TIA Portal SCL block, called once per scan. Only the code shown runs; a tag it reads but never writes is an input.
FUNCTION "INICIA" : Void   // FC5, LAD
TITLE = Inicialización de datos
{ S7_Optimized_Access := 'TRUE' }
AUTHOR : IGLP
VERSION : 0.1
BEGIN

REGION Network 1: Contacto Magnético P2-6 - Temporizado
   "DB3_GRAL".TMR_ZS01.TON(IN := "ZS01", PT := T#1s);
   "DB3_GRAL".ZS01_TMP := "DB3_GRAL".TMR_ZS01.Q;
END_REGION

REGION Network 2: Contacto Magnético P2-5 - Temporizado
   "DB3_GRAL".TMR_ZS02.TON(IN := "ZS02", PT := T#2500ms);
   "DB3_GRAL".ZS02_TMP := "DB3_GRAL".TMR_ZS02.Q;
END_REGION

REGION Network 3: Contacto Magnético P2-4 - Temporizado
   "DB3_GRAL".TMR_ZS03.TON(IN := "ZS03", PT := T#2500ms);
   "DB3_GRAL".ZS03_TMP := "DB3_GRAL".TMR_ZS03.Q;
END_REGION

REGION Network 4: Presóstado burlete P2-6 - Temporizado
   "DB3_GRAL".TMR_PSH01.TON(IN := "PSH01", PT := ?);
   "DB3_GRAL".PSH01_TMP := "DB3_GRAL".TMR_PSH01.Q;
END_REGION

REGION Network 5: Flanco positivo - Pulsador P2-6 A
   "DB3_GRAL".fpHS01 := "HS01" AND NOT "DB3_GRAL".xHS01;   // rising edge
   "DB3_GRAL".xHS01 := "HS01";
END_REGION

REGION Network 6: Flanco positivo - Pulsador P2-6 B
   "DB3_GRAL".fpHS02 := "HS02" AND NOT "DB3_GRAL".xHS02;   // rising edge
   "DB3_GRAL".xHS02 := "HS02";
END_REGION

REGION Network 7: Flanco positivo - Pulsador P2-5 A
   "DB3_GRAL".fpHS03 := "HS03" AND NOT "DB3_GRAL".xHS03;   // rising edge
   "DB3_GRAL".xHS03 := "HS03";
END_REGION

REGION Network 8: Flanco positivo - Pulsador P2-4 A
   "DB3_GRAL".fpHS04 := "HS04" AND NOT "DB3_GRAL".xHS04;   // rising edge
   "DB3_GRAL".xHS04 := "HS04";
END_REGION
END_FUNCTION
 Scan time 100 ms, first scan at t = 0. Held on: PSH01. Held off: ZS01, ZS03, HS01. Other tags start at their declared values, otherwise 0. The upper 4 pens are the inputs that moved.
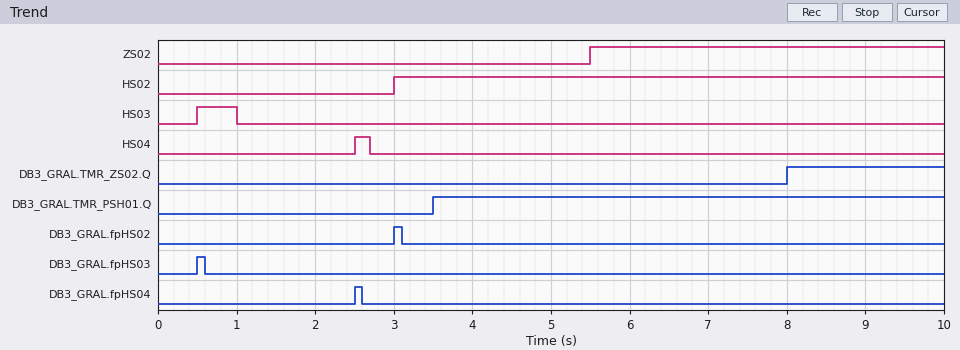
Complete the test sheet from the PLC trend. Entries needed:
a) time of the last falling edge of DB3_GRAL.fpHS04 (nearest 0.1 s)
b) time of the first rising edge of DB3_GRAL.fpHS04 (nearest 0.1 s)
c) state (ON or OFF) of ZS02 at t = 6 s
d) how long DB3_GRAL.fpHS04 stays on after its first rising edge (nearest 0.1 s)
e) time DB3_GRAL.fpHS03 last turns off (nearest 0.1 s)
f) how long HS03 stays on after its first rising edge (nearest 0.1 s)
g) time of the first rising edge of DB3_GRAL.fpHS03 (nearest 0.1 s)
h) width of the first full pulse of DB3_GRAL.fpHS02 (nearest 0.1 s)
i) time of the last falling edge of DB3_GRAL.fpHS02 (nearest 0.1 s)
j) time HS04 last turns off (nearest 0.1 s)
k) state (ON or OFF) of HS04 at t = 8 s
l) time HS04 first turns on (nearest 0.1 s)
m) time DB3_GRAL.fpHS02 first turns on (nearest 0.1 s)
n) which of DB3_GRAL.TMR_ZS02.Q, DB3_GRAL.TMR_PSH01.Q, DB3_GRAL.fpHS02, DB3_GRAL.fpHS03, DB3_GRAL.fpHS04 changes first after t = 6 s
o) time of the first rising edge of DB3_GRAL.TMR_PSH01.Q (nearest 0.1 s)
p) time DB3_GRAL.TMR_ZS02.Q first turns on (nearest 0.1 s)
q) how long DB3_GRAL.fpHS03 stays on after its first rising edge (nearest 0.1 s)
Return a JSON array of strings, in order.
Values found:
["2.6 s", "2.5 s", "ON", "0.1 s", "0.6 s", "0.5 s", "0.5 s", "0.1 s", "3.1 s", "2.7 s", "OFF", "2.5 s", "3.0 s", "DB3_GRAL.TMR_ZS02.Q", "3.5 s", "8.0 s", "0.1 s"]
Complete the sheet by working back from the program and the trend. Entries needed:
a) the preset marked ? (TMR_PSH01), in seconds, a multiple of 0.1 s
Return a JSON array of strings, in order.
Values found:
["3.5 s"]
